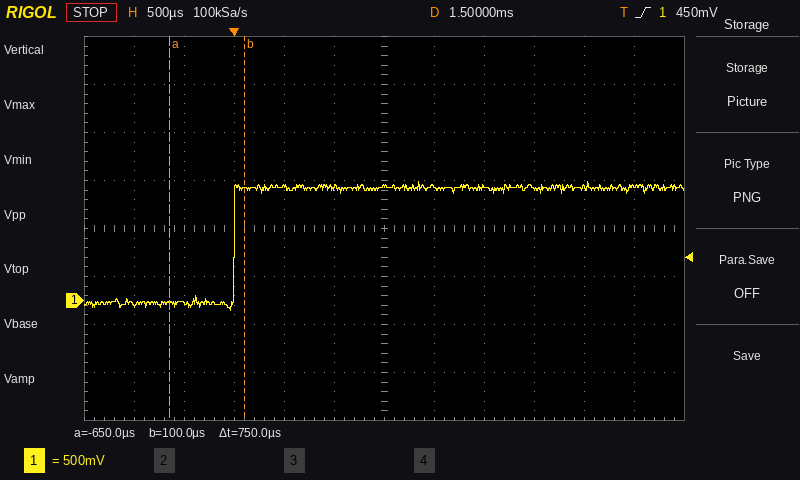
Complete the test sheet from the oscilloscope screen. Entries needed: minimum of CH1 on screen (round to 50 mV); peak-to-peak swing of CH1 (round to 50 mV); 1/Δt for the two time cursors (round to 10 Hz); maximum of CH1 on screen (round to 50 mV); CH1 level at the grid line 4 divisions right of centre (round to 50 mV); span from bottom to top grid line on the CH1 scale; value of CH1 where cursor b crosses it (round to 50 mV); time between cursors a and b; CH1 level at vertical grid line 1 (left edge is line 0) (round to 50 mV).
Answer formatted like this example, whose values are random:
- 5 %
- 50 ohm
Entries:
- -100 mV
- 1.35 V
- 1.33 kHz
- 1.25 V
- 1.20 V
- 4 V
- 1.15 V
- 750 µs
- -50 mV
